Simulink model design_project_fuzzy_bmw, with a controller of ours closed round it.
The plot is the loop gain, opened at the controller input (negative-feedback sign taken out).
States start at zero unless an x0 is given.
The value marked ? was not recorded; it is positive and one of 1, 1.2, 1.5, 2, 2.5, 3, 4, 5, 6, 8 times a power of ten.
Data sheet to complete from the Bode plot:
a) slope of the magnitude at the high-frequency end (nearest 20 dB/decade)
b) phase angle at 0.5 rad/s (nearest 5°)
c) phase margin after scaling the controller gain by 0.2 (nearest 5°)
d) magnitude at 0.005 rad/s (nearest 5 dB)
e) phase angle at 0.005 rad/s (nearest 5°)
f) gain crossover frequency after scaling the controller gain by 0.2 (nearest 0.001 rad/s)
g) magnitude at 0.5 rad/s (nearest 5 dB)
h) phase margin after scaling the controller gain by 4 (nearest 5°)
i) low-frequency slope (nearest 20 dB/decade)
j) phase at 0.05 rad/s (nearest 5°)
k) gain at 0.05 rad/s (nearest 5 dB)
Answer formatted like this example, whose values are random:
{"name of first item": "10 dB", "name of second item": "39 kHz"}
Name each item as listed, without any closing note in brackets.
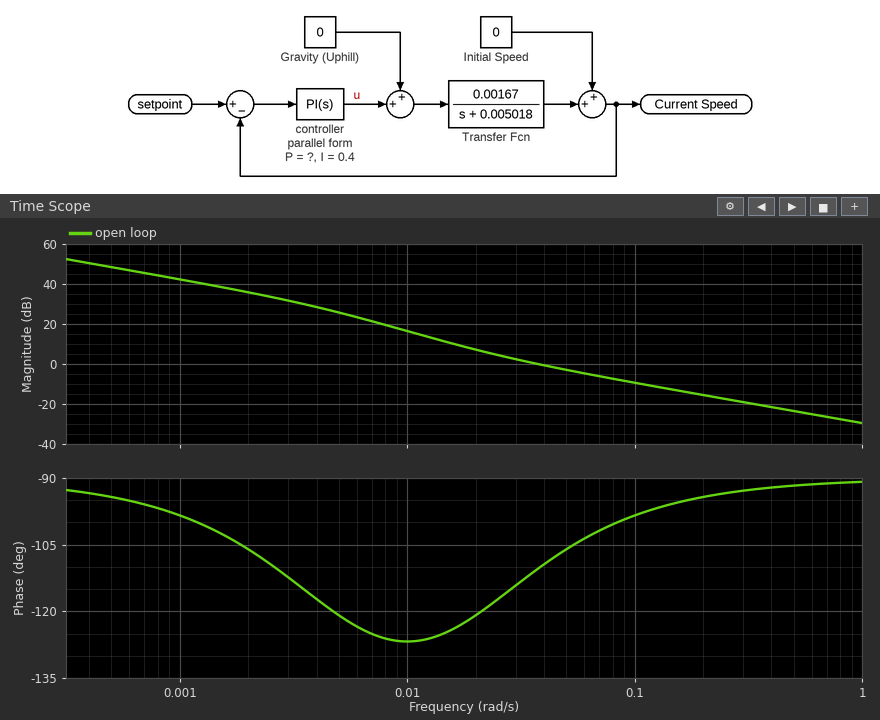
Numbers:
{"slope of the magnitude at the high-frequency end": "-20 dB/decade", "phase angle at 0.5 rad/s": "-90°", "phase margin after scaling the controller gain by 0.2": "55°", "magnitude at 0.005 rad/s": "25 dB", "phase angle at 0.005 rad/s": "-120°", "gain crossover frequency after scaling the controller gain by 0.2": "0.012 rad/s", "magnitude at 0.5 rad/s": "-25 dB", "phase margin after scaling the controller gain by 4": "85°", "low-frequency slope": "-20 dB/decade", "phase at 0.05 rad/s": "-105°", "gain at 0.05 rad/s": "-5 dB"}
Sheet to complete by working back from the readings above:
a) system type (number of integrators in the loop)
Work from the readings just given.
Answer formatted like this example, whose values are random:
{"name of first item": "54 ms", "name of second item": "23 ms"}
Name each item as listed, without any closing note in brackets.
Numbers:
{"system type": "1"}
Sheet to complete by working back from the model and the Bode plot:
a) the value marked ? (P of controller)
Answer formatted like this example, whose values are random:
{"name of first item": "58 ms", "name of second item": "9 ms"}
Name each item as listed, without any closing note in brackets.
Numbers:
{"the value marked ?": "20"}
